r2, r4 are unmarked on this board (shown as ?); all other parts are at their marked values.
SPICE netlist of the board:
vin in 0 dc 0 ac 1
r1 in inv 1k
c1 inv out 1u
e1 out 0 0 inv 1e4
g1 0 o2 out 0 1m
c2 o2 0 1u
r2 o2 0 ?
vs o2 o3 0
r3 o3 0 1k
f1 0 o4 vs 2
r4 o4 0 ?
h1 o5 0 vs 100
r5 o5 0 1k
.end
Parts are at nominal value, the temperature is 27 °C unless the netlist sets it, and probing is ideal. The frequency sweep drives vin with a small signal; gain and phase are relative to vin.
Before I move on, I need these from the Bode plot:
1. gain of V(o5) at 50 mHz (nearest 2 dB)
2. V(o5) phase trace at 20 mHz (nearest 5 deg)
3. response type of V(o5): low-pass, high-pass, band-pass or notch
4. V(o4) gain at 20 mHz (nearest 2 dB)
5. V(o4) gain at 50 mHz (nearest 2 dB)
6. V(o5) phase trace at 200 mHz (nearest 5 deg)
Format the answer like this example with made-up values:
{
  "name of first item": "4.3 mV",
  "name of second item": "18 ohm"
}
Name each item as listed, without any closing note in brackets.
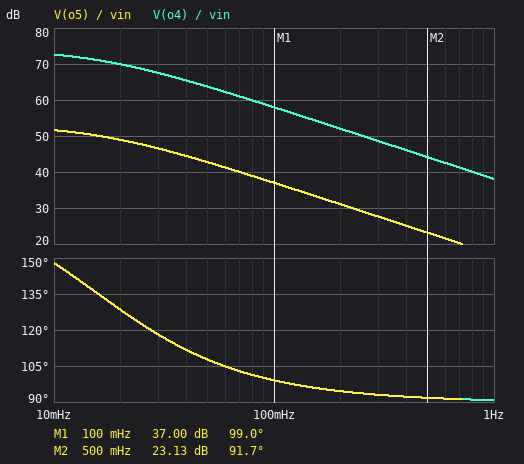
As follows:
{
  "gain of V(o5) at 50 mHz": "42 dB",
  "V(o5) phase trace at 20 mHz": "130 deg",
  "response type of V(o5): low-pass, high-pass, band-pass or notch": "low-pass",
  "V(o4) gain at 20 mHz": "70 dB",
  "V(o4) gain at 50 mHz": "64 dB",
  "V(o5) phase trace at 200 mHz": "95 deg"
}
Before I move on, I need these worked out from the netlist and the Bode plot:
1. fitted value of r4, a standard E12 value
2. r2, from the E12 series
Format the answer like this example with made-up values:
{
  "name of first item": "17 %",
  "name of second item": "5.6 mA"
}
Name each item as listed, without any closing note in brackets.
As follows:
{
  "fitted value of r4, a standard E12 value": "560 Ω",
  "r2, from the E12 series": "820 Ω"
}
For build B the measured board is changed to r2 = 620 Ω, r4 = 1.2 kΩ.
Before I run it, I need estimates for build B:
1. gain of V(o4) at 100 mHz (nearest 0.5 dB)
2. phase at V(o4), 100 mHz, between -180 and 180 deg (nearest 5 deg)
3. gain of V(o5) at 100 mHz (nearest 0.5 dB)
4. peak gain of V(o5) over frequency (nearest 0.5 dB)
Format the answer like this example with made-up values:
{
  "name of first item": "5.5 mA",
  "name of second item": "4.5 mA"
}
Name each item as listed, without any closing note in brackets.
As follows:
{
  "gain of V(o4) at 100 mHz": "63.0 dB",
  "phase at V(o4), 100 mHz, between -180 and 180 deg": "100 deg",
  "gain of V(o5) at 100 mHz": "35.5 dB",
  "peak gain of V(o5) over frequency": "51.5 dB"
}
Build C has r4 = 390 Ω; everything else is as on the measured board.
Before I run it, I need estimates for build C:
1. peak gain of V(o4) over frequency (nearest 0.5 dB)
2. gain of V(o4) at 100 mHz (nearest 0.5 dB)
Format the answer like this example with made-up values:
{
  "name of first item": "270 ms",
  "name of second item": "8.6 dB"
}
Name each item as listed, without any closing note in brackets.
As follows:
{
  "peak gain of V(o4) over frequency": "71.0 dB",
  "gain of V(o4) at 100 mHz": "55.0 dB"
}
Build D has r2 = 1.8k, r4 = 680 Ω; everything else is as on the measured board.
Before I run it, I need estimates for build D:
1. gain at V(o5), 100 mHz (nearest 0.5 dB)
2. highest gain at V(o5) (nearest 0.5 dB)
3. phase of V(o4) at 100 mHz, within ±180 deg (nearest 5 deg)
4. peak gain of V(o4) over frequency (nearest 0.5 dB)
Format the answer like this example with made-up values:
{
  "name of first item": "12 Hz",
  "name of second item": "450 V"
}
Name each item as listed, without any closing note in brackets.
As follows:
{
  "gain at V(o5), 100 mHz": "40.0 dB",
  "highest gain at V(o5)": "56.0 dB",
  "phase of V(o4) at 100 mHz, within ±180 deg": "100 deg",
  "peak gain of V(o4) over frequency": "79.0 dB"
}
